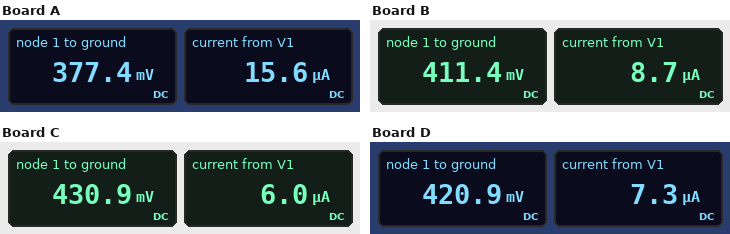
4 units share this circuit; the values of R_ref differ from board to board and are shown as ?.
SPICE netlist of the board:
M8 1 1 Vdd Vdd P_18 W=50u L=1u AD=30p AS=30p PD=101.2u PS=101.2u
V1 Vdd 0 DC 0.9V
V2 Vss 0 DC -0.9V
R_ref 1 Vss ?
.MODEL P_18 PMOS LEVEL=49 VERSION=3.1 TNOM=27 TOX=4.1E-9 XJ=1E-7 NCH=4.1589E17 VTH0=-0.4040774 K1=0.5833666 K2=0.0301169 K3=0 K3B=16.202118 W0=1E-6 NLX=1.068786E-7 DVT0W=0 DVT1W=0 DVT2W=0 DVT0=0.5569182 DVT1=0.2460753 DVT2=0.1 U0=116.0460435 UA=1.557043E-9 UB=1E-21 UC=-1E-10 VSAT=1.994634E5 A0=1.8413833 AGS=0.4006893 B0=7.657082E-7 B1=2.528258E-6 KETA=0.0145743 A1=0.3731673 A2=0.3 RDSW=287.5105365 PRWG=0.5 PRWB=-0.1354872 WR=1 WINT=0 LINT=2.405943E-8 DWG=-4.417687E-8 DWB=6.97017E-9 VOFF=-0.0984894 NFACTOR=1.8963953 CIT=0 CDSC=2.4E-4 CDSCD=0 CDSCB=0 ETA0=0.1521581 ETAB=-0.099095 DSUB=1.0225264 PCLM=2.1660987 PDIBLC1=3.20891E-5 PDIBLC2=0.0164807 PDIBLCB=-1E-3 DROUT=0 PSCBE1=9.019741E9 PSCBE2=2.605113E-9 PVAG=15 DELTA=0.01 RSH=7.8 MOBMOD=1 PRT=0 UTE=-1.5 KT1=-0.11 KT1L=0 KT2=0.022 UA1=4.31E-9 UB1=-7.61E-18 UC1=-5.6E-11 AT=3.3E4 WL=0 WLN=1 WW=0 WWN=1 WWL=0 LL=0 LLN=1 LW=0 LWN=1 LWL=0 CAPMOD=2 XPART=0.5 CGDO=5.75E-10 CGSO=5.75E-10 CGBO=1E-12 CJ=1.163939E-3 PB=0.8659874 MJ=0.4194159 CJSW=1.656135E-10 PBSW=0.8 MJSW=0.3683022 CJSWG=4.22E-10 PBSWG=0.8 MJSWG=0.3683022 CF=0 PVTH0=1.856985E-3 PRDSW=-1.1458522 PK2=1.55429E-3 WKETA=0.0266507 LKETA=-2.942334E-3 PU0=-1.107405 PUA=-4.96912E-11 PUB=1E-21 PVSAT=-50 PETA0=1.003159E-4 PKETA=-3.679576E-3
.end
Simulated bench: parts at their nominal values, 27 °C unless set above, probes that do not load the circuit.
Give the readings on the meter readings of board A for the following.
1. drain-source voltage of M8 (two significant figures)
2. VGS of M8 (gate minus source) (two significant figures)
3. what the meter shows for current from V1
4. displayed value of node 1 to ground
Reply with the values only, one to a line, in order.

-520 mV
-520 mV
15.6 µA
377.4 mV
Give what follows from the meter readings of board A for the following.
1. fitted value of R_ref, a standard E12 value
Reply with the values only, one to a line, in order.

82 kΩ
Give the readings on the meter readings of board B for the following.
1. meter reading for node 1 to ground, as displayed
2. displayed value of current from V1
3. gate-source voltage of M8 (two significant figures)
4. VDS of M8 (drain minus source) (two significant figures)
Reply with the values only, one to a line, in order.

411.4 mV
8.7 µA
-490 mV
-490 mV
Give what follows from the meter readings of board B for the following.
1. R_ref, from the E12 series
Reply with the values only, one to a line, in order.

150 kΩ
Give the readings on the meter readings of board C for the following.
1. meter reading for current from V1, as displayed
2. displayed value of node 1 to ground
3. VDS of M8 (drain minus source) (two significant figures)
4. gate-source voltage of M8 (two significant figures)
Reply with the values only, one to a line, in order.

6.0 µA
430.9 mV
-470 mV
-470 mV
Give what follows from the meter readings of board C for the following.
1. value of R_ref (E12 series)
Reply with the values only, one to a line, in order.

220 kΩ
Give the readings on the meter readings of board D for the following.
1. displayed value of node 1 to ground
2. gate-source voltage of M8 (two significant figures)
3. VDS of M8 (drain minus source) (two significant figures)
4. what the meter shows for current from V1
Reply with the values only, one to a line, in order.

420.9 mV
-480 mV
-480 mV
7.3 µA
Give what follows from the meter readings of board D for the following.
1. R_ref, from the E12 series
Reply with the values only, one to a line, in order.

180 kΩ
